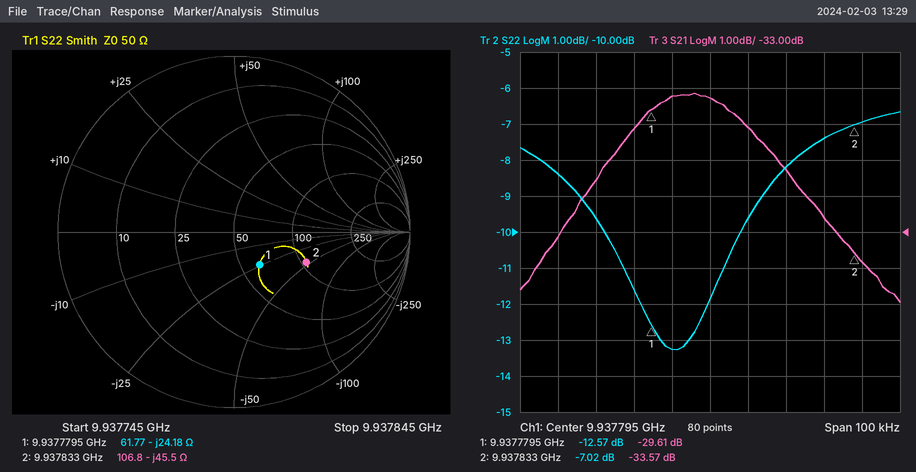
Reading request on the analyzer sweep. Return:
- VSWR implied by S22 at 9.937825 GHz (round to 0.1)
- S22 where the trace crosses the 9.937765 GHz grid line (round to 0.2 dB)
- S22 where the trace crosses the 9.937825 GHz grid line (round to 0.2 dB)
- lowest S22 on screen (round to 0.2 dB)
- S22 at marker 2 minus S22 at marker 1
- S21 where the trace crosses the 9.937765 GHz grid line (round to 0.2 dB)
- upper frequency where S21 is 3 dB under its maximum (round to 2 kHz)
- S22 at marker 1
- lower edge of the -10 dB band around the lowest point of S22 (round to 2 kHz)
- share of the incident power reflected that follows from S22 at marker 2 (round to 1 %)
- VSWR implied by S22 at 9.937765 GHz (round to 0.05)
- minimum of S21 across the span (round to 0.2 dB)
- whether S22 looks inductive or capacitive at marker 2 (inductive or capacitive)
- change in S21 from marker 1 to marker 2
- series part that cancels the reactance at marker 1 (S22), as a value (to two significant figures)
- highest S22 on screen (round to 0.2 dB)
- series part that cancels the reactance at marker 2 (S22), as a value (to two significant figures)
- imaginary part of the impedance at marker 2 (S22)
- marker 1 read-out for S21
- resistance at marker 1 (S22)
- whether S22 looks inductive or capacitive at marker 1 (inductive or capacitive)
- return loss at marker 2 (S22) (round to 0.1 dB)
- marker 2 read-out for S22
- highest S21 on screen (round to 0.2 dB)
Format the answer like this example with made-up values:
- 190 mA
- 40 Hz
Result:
- 2.5
- -9.6 dB
- -7.4 dB
- -13.2 dB
- 5.55 dB
- -31.6 dB
- 9.937822 GHz
- -12.57 dB
- 9.937768 GHz
- 20 %
- 2.00
- -35.0 dB
- capacitive
- -3.96 dB
- 390 pH
- -6.6 dB
- 730 pH
- -45.5 Ω
- -29.61 dB
- 61.77 Ω
- capacitive
- 7.0 dB
- -7.02 dB
- -29.2 dB
